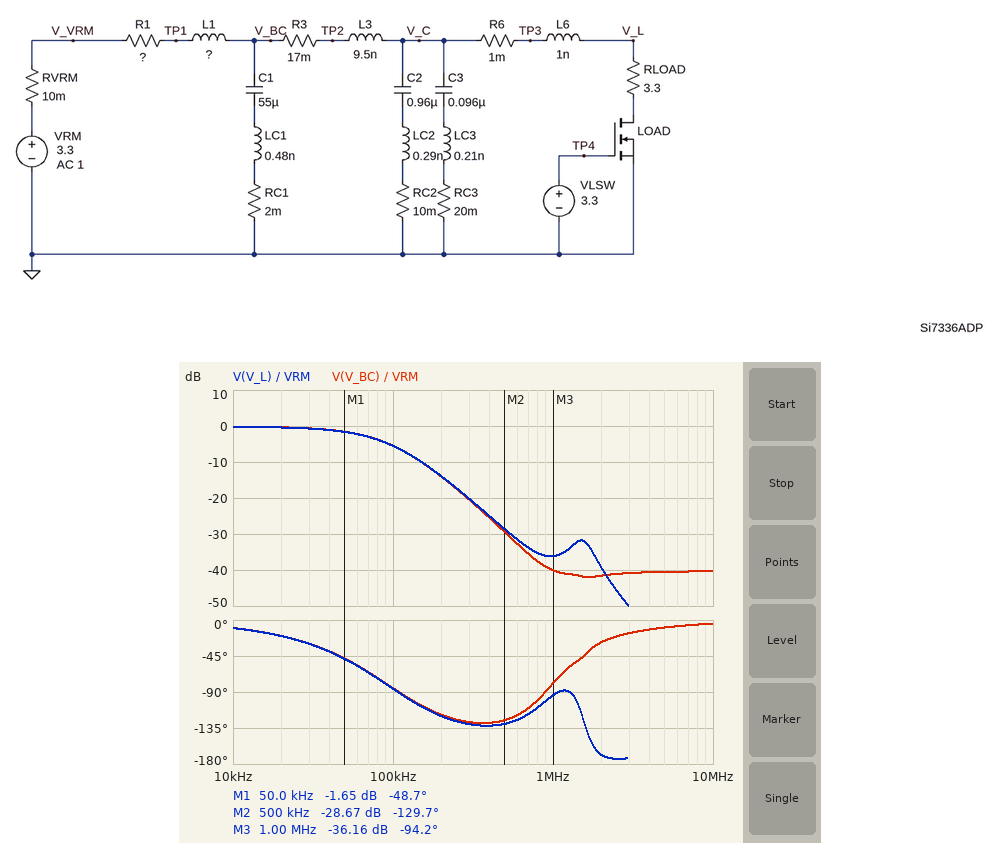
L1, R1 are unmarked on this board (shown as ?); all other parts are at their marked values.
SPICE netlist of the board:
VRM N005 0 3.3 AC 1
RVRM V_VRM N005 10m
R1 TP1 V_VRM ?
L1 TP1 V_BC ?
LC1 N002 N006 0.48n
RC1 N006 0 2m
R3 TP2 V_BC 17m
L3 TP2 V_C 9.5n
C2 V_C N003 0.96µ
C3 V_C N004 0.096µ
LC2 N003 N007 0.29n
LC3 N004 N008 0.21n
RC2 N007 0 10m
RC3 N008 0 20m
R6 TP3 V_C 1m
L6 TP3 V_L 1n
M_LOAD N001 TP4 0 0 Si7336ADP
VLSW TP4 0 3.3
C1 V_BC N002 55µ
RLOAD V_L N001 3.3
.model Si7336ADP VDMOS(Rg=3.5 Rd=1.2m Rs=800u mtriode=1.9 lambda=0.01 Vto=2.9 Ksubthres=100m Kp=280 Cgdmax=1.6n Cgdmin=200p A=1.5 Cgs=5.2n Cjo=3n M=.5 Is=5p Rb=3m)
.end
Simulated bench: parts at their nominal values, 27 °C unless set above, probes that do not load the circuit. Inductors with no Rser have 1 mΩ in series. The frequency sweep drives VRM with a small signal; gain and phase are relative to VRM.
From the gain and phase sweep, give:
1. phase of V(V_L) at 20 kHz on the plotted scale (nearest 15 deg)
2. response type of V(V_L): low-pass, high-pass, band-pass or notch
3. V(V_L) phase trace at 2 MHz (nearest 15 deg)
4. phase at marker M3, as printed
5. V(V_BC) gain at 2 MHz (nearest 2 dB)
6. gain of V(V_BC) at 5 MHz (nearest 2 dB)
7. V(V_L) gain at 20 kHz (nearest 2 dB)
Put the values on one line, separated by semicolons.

-15 deg; low-pass; -165 deg; -94.2 deg; -42 dB; -40 dB; 0 dB
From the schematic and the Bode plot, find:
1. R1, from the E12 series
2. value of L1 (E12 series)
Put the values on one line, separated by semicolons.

0.039 Ω; 47 nH
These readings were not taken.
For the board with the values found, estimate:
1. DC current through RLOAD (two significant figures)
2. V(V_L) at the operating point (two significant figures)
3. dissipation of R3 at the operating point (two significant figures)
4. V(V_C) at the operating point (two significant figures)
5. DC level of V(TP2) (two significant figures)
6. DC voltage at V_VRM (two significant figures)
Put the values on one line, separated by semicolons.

980 mA; 3.2 V; 16 mW; 3.2 V; 3.2 V; 3.3 V
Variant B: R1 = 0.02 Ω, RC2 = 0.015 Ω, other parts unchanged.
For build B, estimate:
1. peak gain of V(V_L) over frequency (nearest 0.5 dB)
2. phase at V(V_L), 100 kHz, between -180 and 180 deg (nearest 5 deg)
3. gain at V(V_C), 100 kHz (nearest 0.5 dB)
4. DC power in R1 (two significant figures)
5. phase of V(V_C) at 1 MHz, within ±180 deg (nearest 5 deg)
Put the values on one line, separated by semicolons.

0.5 dB; -85 deg; -1.5 dB; 19 mW; -100 deg
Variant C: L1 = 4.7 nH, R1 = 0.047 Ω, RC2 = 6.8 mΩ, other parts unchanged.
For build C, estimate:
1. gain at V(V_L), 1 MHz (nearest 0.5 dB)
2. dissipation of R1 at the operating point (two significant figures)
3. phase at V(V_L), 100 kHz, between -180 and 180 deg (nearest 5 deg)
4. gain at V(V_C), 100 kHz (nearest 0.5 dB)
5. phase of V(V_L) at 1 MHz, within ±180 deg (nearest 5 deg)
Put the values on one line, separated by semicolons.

-23.0 dB; 45 mW; -60 deg; -7.5 dB; -40 deg
